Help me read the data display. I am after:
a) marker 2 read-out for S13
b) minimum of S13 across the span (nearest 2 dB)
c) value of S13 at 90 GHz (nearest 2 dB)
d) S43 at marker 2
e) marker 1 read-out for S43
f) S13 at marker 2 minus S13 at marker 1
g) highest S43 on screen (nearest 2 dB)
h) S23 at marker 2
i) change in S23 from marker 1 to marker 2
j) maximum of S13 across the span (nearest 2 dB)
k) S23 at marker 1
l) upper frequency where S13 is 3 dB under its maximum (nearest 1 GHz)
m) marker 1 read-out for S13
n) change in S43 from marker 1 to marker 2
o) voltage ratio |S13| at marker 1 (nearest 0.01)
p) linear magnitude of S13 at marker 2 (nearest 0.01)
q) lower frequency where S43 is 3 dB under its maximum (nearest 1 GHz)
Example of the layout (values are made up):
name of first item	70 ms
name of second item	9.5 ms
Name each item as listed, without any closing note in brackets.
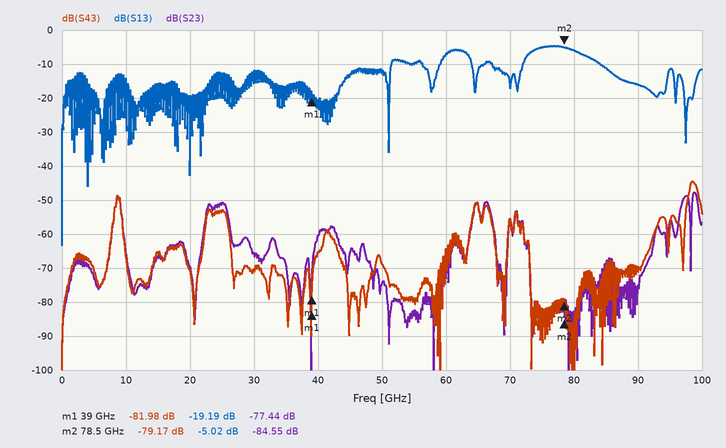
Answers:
marker 2 read-out for S13	-5.02 dB
minimum of S13 across the span	-64 dB
value of S13 at 90 GHz	-16 dB
S43 at marker 2	-79.17 dB
marker 1 read-out for S43	-81.98 dB
S13 at marker 2 minus S13 at marker 1	14.17 dB
highest S43 on screen	-44 dB
S23 at marker 2	-84.55 dB
change in S23 from marker 1 to marker 2	-7.11 dB
maximum of S13 across the span	-4 dB
S23 at marker 1	-77.44 dB
upper frequency where S13 is 3 dB under its maximum	82 GHz
marker 1 read-out for S13	-19.19 dB
change in S43 from marker 1 to marker 2	2.81 dB
voltage ratio |S13| at marker 1	0.11
linear magnitude of S13 at marker 2	0.56
lower frequency where S43 is 3 dB under its maximum	98 GHz
